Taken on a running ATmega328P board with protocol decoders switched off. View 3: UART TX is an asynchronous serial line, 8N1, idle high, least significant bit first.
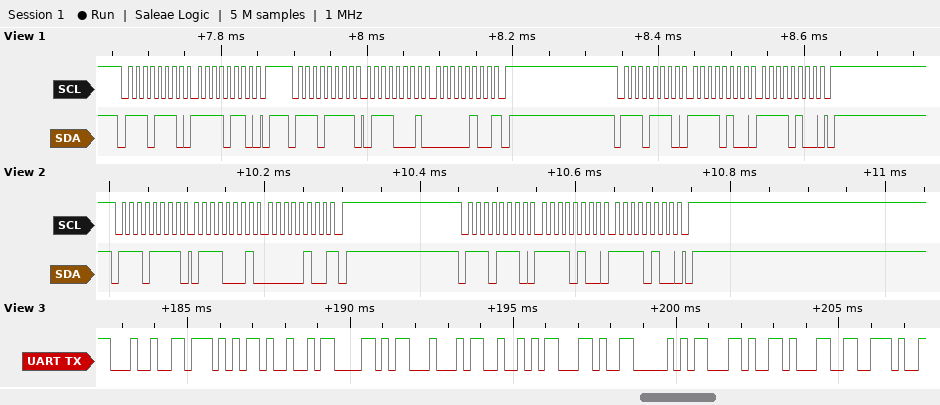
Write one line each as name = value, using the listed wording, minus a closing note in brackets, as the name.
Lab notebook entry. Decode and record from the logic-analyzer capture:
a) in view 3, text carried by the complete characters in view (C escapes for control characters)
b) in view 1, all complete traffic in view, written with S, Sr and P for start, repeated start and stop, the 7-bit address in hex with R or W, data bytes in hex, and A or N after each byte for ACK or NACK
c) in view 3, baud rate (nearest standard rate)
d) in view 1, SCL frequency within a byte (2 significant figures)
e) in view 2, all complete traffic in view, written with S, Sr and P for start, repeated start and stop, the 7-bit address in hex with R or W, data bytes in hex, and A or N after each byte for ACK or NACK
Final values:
in view 3, text carried by the complete characters in view = "$WIXDR,P,1."
in view 1, all complete traffic in view, written with S, Sr and P for start, repeated start and stop, the 7-bit address in hex with R or W, data bytes in hex, and A or N after each byte for ACK or NACK = S 77W A F6 A P S 77R A 71 A 04 N P S 77W A F4 A F4 A P
in view 3, baud rate = 4800 baud
in view 1, SCL frequency within a byte = 100 kHz
in view 2, all complete traffic in view, written with S, Sr and P for start, repeated start and stop, the 7-bit address in hex with R or W, data bytes in hex, and A or N after each byte for ACK or NACK = S 77R A 71 A 04 N P S 77W A F4 A F4 A P
